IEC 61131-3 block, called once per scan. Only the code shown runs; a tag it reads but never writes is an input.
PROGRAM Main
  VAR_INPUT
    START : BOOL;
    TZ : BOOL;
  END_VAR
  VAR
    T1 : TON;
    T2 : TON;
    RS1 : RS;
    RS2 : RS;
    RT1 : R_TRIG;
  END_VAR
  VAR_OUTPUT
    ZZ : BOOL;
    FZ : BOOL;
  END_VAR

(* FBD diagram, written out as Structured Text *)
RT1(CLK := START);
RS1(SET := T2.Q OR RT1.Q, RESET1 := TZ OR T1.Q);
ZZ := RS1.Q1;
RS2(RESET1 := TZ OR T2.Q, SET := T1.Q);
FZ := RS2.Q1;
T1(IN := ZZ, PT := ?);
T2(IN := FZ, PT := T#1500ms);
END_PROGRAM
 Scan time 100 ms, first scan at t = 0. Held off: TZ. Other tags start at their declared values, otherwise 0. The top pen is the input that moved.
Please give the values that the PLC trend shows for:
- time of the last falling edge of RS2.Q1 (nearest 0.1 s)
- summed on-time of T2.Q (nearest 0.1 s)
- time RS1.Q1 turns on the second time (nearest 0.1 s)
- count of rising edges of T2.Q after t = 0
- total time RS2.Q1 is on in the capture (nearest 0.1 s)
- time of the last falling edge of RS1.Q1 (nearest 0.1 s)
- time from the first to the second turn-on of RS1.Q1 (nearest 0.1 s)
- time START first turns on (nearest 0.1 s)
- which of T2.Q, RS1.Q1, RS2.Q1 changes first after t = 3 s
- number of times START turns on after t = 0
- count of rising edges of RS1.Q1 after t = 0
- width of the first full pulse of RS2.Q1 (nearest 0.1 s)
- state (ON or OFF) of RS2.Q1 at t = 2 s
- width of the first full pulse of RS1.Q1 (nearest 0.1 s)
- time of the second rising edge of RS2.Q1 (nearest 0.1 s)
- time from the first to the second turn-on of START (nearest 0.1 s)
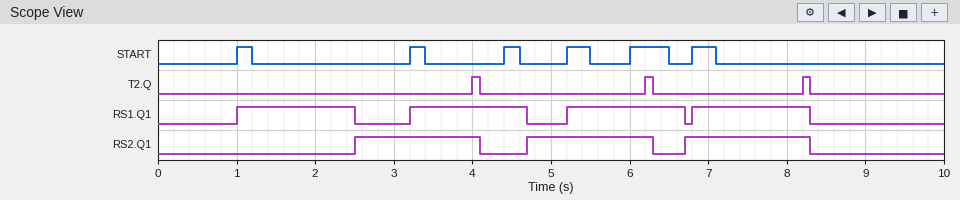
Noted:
8.3 s
0.3 s
3.2 s
3
4.8 s
8.3 s
2.2 s
1.0 s
RS1.Q1
6
4
1.6 s
OFF
1.5 s
4.7 s
2.2 s
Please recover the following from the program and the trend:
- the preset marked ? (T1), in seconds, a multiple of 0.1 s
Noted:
1.4 s
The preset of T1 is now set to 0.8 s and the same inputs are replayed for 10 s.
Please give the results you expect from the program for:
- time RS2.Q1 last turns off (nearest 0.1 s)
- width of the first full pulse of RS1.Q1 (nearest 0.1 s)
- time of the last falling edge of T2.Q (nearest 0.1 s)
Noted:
8.2 s
0.9 s
8.2 s
